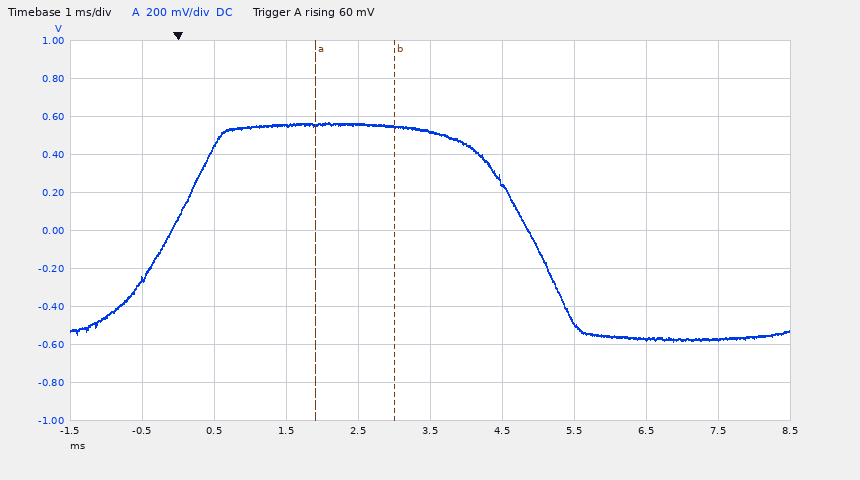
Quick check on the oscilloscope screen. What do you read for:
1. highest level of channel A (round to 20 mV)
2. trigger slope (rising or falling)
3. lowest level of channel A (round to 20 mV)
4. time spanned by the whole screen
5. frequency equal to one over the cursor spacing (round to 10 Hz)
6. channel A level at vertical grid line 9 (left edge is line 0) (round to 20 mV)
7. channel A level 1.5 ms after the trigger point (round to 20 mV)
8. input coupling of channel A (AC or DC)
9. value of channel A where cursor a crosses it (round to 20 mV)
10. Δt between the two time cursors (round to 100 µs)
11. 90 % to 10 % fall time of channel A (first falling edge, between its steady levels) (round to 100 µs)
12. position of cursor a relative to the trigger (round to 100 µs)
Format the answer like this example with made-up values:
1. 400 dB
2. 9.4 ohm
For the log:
1. 560 mV
2. rising
3. -580 mV
4. 10 ms
5. 910 Hz
6. -580 mV
7. 560 mV
8. DC
9. 560 mV
10. 1.1 ms
11. 1.4 ms
12. +1.9 ms
